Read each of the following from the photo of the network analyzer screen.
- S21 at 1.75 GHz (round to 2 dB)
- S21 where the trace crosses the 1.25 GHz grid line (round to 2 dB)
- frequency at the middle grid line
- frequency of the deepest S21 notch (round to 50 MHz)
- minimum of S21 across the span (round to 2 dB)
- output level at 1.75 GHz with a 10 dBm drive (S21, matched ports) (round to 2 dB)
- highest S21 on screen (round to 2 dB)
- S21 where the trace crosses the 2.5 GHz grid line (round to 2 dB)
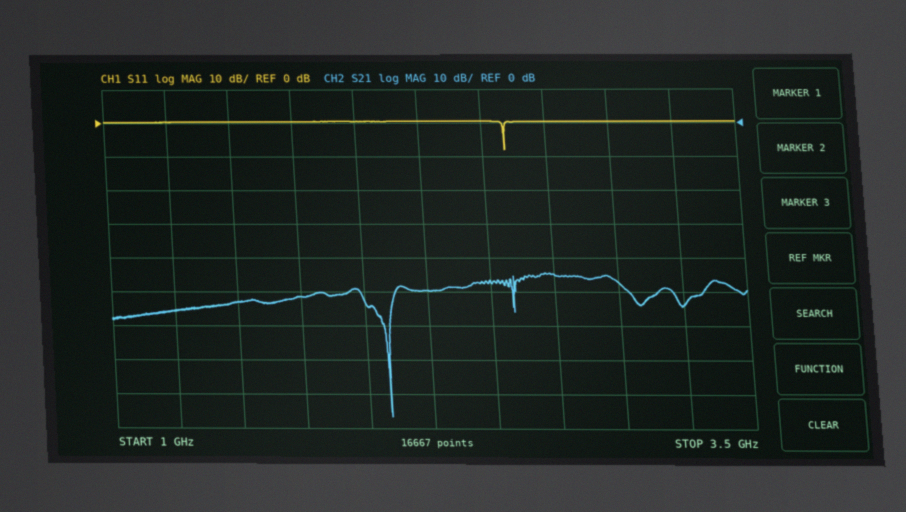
-52 dB
-56 dB
2.25 GHz
2.10 GHz
-86 dB
-42 dBm
-44 dB
-46 dB
